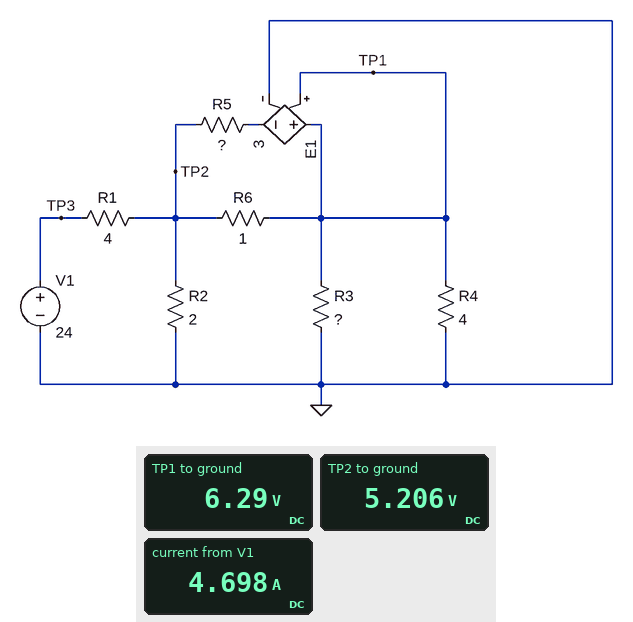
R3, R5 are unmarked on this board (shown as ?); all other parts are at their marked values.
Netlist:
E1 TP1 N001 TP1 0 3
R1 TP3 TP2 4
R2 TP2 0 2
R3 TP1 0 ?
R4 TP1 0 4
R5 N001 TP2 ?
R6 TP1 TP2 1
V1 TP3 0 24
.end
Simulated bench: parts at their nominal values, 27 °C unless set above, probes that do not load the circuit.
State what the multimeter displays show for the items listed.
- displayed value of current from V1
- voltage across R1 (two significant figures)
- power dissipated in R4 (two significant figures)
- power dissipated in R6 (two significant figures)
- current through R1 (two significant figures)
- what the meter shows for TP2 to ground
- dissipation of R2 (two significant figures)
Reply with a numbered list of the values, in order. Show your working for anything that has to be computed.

1. 4.698 A
2. 24 V - 5.206 V = 19 V
3. (6.29 V)^2 / 4 Ω = 9.9 W
4. (6.29 V - 5.206 V)^2 / 1 Ω = 1.2 W
5. (24 V - 5.206 V) / 4 Ω = 4.7 A
6. 5.206 V
7. (5.206 V)^2 / 2 Ω = 14 W
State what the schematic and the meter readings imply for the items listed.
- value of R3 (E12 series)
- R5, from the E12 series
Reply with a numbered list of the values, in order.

1. 12 Ω
2. 5.6 Ω
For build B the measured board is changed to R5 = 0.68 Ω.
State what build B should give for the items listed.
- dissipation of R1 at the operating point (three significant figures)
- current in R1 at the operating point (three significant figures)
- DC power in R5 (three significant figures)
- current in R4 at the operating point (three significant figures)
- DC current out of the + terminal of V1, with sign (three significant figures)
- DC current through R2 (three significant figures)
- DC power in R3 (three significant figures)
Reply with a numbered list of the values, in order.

1. 379 mW
2. 308 mA
3. 4.02 kW
4. 9.69 A
5. -308 mA
6. 12.6 A
7. 125 W
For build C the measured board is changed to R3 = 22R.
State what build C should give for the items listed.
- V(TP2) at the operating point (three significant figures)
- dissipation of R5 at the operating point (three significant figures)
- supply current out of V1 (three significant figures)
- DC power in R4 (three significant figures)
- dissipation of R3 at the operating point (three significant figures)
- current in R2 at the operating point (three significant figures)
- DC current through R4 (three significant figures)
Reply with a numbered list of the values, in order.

1. 5.35 V
2. 63.1 W
3. 4.66 A
4. 11.3 W
5. 2.05 W
6. 2.68 A
7. 1.68 A
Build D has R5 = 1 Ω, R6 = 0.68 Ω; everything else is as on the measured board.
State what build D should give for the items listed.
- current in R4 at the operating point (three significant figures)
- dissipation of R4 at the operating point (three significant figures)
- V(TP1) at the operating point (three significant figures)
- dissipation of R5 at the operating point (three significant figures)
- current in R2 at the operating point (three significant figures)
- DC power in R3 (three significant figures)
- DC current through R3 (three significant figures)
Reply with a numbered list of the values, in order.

1. 5.48 A
2. 120 W
3. 21.9 V
4. 1.77 kW
5. 870 mA
6. 40.0 W
7. 1.83 A
